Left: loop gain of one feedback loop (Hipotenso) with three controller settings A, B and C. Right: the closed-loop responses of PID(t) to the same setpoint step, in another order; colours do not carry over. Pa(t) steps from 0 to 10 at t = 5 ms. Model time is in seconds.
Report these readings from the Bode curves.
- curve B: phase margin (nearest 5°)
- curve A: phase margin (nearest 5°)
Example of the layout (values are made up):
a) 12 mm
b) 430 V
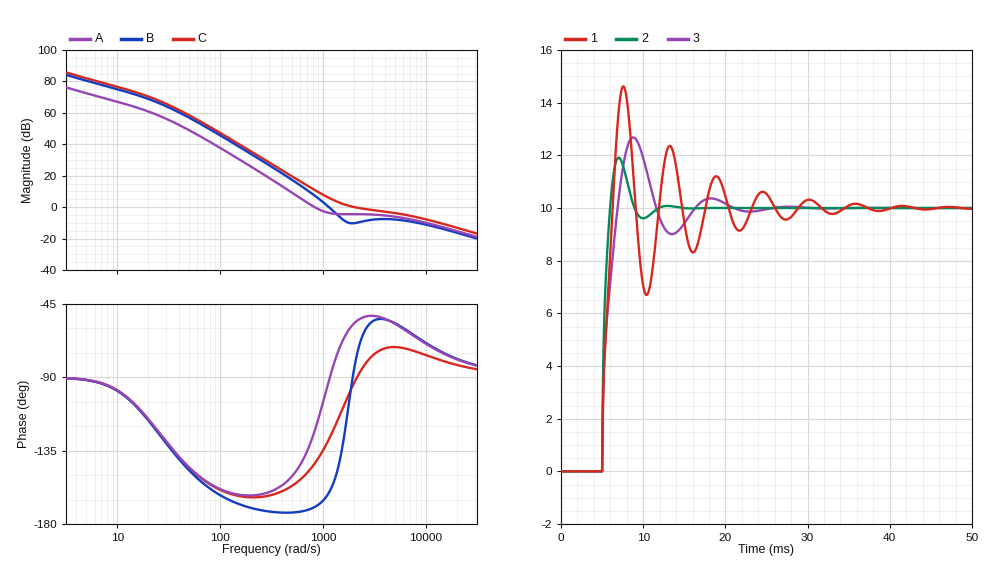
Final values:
a) 20°
b) 55°
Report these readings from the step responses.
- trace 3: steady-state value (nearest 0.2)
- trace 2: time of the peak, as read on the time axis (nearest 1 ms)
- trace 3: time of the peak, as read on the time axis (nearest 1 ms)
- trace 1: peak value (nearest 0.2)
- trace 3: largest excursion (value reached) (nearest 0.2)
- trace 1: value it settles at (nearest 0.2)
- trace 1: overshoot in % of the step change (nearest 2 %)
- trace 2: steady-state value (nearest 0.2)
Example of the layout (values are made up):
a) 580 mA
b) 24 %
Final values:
a) 10.0
b) 7 ms
c) 9 ms
d) 14.6
e) 12.6
f) 10.0
g) 46 %
h) 10.0
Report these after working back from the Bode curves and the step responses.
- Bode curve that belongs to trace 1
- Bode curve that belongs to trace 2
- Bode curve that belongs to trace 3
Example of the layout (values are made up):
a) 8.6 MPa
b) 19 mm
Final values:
a) B
b) C
c) A
